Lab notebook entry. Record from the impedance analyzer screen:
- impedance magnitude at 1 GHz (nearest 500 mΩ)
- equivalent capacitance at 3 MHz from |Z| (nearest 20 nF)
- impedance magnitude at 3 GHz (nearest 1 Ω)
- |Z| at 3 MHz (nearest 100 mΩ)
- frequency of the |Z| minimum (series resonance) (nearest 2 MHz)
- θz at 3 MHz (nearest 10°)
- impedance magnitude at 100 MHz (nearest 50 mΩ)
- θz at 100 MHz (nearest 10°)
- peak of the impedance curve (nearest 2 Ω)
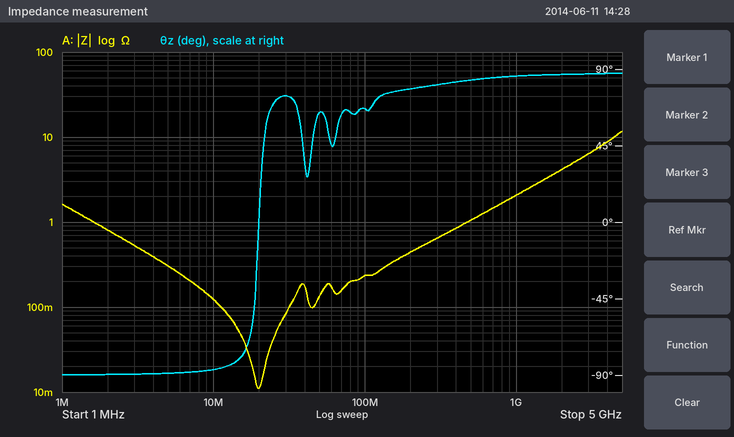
2.0 Ω
100 nF
6 Ω
500 mΩ
20 MHz
-90°
250 mΩ
70°
12 Ω
